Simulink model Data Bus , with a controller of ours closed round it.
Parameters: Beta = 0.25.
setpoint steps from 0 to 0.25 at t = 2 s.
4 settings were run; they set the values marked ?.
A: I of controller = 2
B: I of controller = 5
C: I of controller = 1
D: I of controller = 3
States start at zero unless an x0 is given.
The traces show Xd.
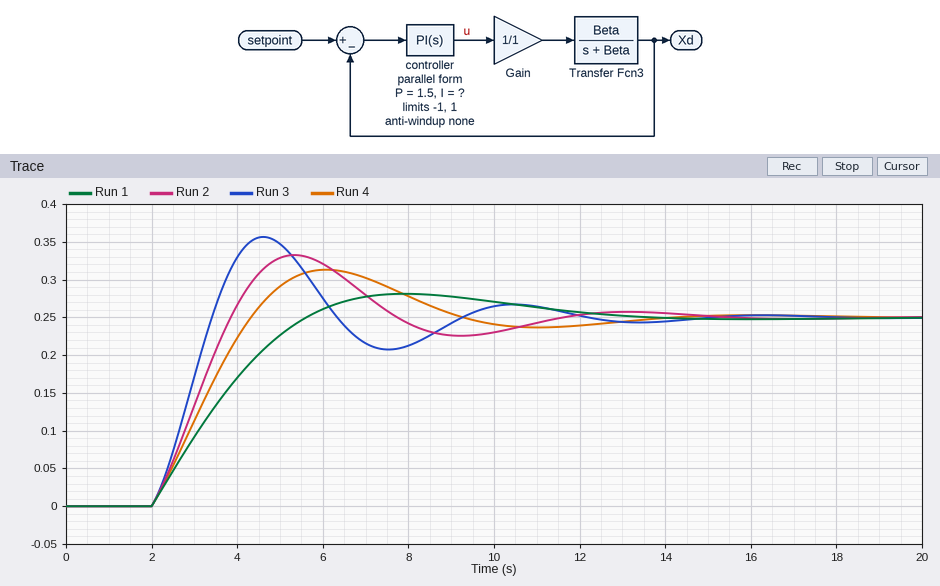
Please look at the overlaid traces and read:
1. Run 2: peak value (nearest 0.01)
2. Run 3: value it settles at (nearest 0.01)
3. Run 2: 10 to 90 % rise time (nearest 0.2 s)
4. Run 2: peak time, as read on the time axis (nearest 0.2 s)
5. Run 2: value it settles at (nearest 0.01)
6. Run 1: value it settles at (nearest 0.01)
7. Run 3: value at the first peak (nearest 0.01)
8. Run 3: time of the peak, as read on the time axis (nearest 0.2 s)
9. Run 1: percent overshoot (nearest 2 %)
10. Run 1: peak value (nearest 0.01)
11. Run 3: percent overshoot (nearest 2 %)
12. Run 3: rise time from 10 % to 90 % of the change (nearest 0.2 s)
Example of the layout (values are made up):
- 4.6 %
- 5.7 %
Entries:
- 0.33
- 0.25
- 1.4 s
- 5.4 s
- 0.25
- 0.25
- 0.36
- 4.6 s
- 12 %
- 0.28
- 42 %
- 1.0 s
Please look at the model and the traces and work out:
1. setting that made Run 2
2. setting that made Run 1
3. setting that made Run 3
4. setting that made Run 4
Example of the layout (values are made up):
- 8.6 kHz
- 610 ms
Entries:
- D
- C
- B
- A
